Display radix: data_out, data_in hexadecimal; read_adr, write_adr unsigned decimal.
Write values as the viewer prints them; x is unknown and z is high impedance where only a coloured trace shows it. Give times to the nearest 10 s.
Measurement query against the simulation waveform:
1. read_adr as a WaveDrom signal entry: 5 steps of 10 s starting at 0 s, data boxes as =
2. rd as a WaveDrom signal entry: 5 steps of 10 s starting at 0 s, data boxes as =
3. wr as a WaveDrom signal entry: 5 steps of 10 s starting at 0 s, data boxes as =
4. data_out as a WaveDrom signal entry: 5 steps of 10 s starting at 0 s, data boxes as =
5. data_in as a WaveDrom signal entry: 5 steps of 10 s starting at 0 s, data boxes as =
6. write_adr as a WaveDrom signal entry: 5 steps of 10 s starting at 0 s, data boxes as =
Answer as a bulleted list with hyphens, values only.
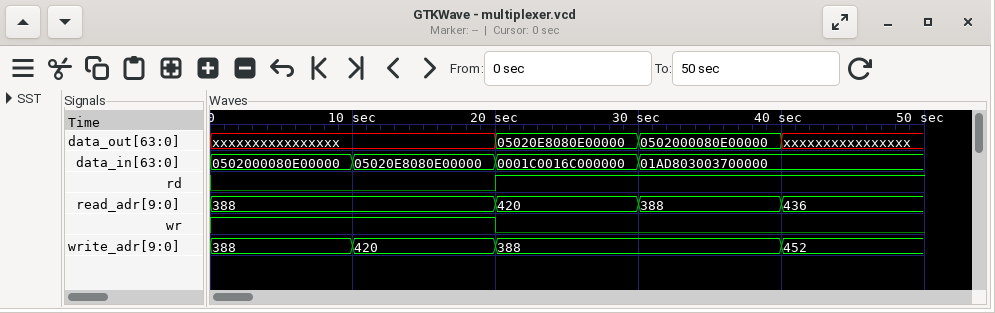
- {name: 'read_adr', wave: '=.===', data: '388 420 388 436'}
- {name: 'rd', wave: '0.1..'}
- {name: 'wr', wave: '1.0..'}
- {name: 'data_out', wave: 'x.==x', data: '05020E8080E00000 0502000080E00000'}
- {name: 'data_in', wave: '====.', data: '0502000080E00000 05020E8080E00000 0001C0016C000000 01AD803003700000'}
- {name: 'write_adr', wave: '===.=', data: '388 420 388 452'}
